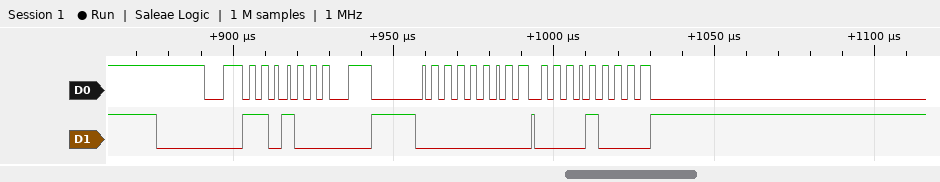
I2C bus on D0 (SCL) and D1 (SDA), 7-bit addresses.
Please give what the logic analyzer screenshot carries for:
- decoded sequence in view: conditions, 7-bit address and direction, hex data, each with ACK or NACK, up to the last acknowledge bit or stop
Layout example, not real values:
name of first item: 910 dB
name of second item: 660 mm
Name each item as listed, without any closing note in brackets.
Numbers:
decoded sequence in view: conditions, 7-bit address and direction, hex data, each with ACK or NACK, up to the last acknowledge bit or stop: start, address 34 write ACK, 00 ACK, 08 ACK
